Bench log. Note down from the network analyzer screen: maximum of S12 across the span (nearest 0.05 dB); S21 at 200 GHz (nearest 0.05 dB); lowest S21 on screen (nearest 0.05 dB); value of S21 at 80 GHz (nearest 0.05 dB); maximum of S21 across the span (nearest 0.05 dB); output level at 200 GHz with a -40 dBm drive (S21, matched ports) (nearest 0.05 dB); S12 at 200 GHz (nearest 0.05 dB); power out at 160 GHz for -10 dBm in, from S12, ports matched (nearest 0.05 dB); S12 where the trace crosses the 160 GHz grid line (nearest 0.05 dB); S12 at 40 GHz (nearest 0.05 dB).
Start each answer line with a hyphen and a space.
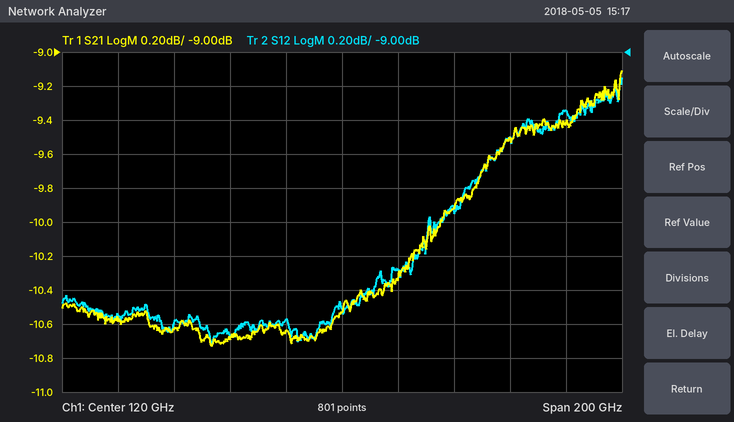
- -9.15 dB
- -9.40 dB
- -10.75 dB
- -10.70 dB
- -9.10 dB
- -49.40 dBm
- -9.35 dB
- -19.95 dBm
- -9.95 dB
- -10.55 dB
